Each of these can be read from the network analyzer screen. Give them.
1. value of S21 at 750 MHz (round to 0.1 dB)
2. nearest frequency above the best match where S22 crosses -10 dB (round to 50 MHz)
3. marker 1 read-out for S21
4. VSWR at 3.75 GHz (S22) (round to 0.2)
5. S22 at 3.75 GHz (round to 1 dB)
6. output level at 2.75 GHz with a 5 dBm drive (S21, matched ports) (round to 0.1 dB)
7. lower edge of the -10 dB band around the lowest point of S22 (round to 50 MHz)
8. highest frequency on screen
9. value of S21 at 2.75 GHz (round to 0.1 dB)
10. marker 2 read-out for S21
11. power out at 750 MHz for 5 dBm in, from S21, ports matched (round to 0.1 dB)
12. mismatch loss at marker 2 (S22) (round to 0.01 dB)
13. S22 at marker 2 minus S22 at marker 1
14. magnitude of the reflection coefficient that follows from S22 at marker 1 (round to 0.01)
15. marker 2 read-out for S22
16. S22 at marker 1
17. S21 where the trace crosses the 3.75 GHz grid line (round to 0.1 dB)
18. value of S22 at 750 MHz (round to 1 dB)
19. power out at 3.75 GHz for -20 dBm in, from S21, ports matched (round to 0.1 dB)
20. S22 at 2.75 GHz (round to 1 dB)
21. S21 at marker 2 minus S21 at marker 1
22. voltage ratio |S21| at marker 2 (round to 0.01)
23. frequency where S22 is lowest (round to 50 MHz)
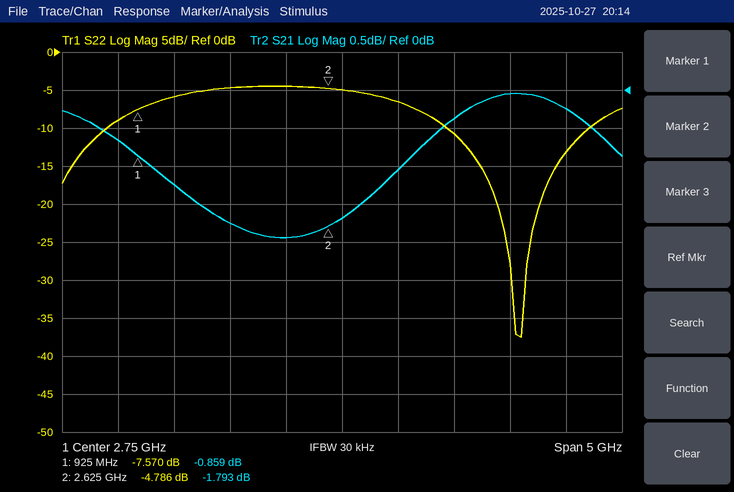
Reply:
-0.7 dB
4.95 GHz
-0.859 dB
1.8
-11 dB
3.3 dBm
3.70 GHz
5.25 GHz
-1.7 dB
-1.793 dB
4.3 dBm
1.75 dB
2.784 dB
0.42
-4.786 dB
-7.570 dB
-0.4 dB
-9 dB
-20.4 dBm
-5 dB
-0.934 dB
0.81
4.35 GHz
